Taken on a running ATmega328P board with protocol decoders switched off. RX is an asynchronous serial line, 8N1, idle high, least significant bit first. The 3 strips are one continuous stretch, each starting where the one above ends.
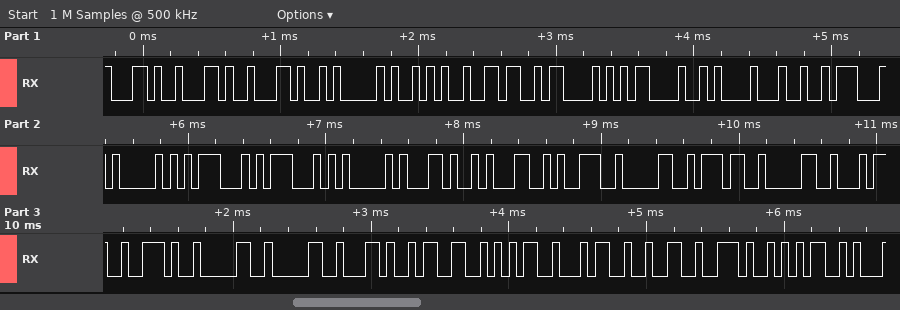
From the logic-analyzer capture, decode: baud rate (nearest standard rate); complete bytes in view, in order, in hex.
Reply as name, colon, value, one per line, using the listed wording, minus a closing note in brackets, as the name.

baud rate: 19200 baud
complete bytes in view, in order, in hex: 2C 2C 2C 41 2A 36 43 0D 0A 24 47 50 47 47 41 2C 31 39 30 37 30 34 2E 30 30 2C 33 35 34 32 2E 35
